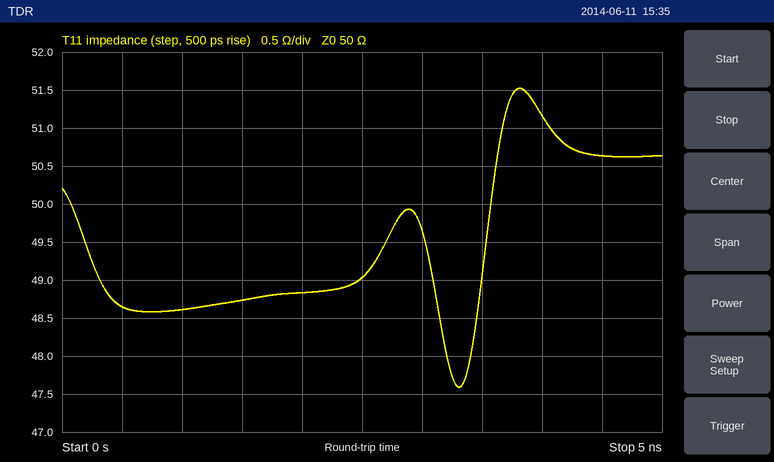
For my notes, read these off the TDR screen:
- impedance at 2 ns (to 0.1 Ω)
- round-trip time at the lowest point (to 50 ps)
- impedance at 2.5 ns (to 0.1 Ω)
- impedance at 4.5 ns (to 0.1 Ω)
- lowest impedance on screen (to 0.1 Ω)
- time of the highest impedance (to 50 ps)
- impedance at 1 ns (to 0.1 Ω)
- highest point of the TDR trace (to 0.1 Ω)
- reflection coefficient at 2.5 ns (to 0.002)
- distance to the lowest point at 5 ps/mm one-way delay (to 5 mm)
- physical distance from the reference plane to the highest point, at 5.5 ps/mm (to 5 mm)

48.8 Ω
3.30 ns
49.0 Ω
50.6 Ω
47.6 Ω
3.80 ns
48.6 Ω
51.5 Ω
-0.010
330 mm
345 mm
